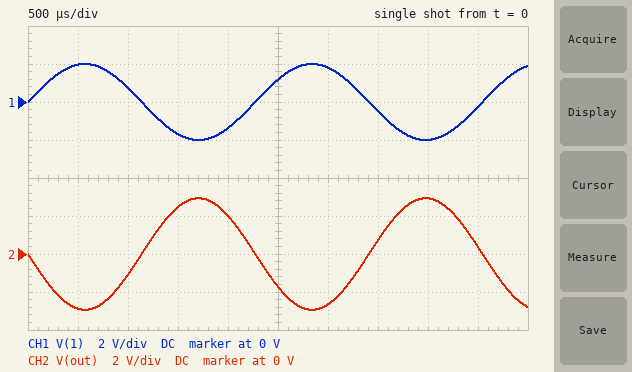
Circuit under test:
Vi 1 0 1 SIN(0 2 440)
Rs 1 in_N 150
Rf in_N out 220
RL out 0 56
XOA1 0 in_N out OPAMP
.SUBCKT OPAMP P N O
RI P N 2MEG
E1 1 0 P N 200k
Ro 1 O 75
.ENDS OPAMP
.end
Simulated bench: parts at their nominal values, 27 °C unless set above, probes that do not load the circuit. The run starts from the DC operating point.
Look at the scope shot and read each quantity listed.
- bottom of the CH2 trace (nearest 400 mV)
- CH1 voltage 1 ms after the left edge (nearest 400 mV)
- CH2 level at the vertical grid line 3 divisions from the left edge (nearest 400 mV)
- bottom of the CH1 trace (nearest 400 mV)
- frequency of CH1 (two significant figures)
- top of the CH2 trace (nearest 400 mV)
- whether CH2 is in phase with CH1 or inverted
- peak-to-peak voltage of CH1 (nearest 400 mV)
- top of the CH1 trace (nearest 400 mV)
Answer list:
-2.8 V
800 mV
2.4 V
-2.0 V
440 Hz
2.8 V
inverted
4.0 V
2.0 V
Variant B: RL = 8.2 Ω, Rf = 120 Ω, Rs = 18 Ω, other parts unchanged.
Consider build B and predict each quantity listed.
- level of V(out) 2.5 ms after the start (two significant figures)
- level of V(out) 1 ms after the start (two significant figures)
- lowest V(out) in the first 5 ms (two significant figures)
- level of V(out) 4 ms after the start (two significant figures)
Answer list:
-7.8 V
-4.9 V
-13 V
13 V
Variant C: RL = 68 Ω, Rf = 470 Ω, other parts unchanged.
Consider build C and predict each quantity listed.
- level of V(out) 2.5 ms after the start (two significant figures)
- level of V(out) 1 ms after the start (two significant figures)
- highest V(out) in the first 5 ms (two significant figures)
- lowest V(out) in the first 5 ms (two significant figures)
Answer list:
-3.7 V
-2.3 V
6.3 V
-6.3 V
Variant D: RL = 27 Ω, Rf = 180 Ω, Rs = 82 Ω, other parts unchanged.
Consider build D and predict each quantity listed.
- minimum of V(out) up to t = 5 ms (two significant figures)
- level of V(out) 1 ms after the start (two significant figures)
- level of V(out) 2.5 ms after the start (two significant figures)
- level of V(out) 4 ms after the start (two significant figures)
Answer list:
-4.4 V
-1.6 V
-2.6 V
4.4 V
